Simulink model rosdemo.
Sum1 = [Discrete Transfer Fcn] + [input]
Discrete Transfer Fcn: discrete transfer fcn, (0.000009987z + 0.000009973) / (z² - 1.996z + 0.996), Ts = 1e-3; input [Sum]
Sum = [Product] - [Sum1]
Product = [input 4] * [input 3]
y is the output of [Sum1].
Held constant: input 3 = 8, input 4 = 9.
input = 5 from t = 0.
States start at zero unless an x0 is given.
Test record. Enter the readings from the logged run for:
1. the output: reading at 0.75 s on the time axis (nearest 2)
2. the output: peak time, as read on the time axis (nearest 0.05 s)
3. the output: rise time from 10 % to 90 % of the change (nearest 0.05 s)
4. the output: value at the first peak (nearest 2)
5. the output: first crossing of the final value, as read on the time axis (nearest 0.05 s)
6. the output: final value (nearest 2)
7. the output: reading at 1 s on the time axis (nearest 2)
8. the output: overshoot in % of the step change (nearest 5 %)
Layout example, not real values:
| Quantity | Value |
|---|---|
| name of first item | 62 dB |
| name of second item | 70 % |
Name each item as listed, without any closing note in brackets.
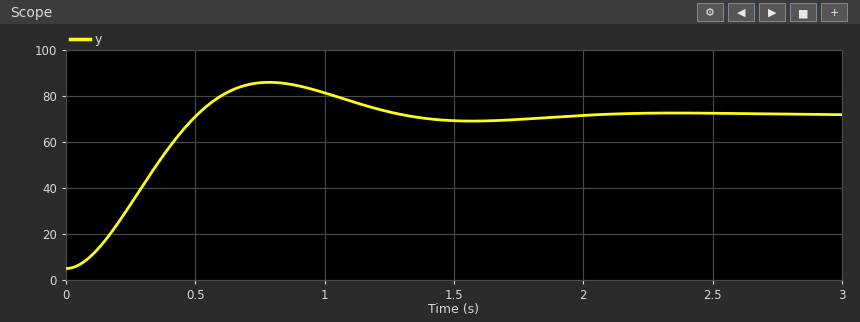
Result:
| Quantity | Value |
|---|---|
| the output: reading at 0.75 s on the time axis | 86 |
| the output: peak time, as read on the time axis | 0.80 s |
| the output: rise time from 10 % to 90 % of the change | 0.35 s |
| the output: value at the first peak | 86 |
| the output: first crossing of the final value, as read on the time axis | 0.50 s |
| the output: final value | 72 |
| the output: reading at 1 s on the time axis | 82 |
| the output: overshoot in % of the step change | 20 % |
